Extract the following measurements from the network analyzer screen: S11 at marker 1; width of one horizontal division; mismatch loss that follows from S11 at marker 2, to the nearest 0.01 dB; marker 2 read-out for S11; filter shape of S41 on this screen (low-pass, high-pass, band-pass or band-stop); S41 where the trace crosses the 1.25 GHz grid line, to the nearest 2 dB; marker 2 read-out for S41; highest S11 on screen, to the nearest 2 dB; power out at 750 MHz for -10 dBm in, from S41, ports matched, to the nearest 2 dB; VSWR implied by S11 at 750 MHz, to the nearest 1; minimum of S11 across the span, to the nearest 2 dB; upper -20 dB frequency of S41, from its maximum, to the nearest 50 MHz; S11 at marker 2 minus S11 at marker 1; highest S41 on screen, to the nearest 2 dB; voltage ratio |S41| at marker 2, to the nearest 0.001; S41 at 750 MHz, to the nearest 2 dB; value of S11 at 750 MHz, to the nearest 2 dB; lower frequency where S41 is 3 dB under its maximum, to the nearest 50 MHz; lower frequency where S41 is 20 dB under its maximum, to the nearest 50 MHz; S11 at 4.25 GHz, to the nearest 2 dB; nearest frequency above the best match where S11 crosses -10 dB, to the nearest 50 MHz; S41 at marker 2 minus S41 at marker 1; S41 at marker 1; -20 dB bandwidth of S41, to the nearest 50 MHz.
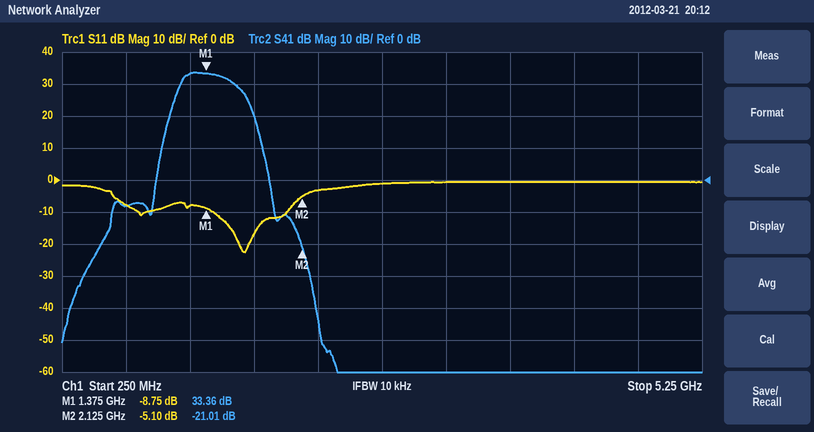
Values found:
-8.75 dB
500 MHz
1.61 dB
-5.10 dB
band-pass
34 dB
-21.01 dB
0 dB
-18 dBm
2
-22 dB
1.80 GHz
3.65 dB
34 dB
0.089
-8 dB
-8 dB
1.20 GHz
1.05 GHz
0 dB
2.00 GHz
-54.37 dB
33.36 dB
750 MHz
